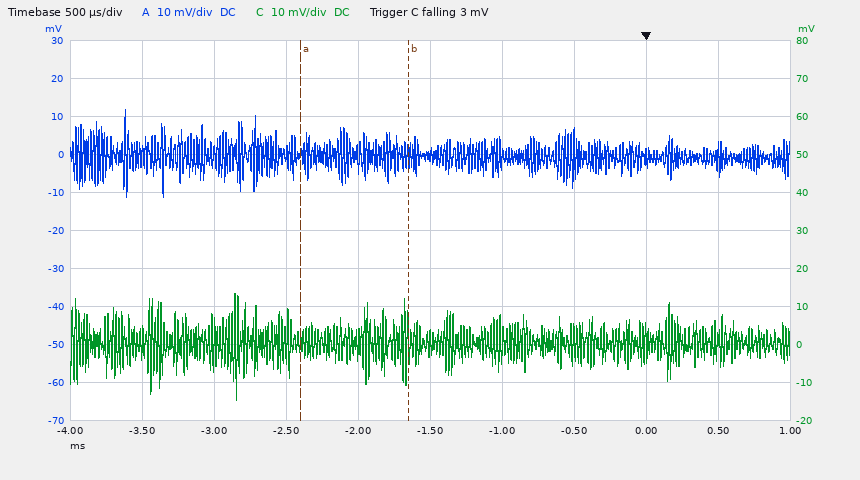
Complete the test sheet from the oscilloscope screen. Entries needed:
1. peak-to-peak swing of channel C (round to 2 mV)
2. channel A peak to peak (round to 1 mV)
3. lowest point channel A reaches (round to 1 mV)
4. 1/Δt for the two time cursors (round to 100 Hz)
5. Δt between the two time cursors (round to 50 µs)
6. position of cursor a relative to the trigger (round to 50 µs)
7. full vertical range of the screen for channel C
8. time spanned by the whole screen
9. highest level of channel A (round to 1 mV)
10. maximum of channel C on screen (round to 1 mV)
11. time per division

28 mV
23 mV
-11 mV
1.3 kHz
750 µs
-2.40 ms
100 mV
5 ms
12 mV
13 mV
500 µs
